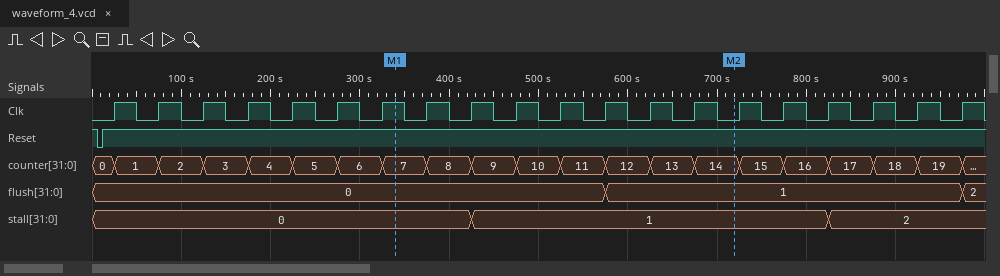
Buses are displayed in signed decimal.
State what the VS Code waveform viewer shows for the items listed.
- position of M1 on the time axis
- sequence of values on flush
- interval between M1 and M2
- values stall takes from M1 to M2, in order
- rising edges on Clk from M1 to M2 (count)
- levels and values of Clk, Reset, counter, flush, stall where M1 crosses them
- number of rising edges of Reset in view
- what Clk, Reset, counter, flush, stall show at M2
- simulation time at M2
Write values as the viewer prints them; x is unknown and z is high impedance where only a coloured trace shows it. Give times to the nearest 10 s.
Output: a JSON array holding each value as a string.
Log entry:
["340 s", "0, 1, 2", "380 s", "0, 1", "7", "Clk=1, Reset=1, counter=7, flush=0, stall=0", "1", "Clk=0, Reset=1, counter=14, flush=1, stall=1", "720 s"]
